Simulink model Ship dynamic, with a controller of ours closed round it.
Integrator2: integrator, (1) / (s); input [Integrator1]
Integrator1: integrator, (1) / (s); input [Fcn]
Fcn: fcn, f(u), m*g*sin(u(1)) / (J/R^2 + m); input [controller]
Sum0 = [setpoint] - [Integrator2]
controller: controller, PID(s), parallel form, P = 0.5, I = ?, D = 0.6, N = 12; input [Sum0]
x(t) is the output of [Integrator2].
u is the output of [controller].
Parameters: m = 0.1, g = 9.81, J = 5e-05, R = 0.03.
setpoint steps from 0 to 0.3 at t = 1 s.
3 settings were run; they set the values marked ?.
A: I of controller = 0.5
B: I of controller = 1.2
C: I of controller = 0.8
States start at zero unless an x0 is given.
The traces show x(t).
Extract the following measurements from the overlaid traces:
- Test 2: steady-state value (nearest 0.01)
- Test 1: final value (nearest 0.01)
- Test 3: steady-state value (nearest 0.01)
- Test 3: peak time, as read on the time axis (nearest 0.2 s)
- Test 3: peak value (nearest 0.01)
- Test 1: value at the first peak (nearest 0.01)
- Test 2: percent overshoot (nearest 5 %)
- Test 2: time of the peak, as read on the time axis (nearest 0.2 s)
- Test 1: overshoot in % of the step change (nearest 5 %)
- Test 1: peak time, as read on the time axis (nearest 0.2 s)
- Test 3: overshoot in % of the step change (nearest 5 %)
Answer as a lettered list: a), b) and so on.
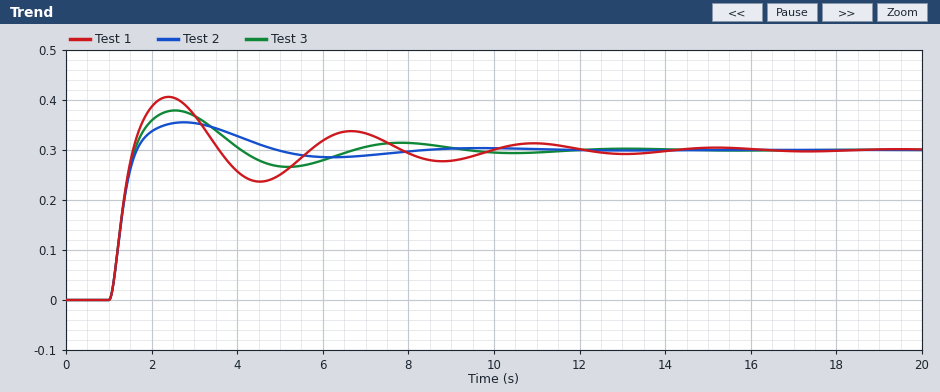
a) 0.30
b) 0.30
c) 0.30
d) 2.6 s
e) 0.38
f) 0.41
g) 20 %
h) 2.8 s
i) 35 %
j) 2.4 s
k) 25 %
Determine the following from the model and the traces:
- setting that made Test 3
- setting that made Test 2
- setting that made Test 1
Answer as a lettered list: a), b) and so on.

a) C
b) A
c) B
